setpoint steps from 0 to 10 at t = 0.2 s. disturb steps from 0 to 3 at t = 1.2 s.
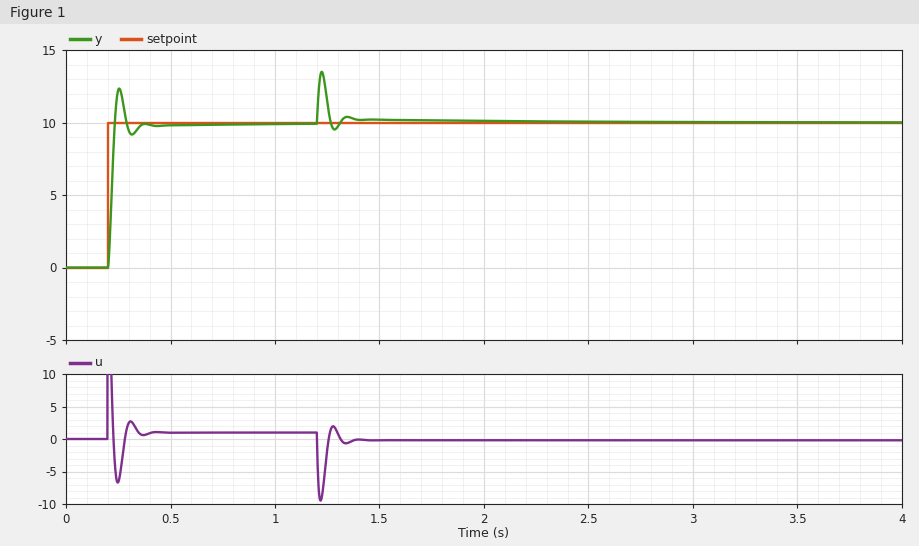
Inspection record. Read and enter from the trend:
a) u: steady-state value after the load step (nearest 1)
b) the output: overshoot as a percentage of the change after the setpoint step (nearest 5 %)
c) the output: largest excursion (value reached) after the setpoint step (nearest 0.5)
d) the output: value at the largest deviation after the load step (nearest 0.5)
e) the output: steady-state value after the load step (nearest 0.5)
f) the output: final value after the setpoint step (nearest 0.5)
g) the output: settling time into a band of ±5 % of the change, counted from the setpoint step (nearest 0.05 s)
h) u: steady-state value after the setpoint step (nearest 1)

0
25 %
12.5
13.5
10.0
10.0
0.15 s
1
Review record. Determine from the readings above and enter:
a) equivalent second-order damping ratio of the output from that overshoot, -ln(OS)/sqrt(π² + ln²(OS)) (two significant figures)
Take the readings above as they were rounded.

0.40
